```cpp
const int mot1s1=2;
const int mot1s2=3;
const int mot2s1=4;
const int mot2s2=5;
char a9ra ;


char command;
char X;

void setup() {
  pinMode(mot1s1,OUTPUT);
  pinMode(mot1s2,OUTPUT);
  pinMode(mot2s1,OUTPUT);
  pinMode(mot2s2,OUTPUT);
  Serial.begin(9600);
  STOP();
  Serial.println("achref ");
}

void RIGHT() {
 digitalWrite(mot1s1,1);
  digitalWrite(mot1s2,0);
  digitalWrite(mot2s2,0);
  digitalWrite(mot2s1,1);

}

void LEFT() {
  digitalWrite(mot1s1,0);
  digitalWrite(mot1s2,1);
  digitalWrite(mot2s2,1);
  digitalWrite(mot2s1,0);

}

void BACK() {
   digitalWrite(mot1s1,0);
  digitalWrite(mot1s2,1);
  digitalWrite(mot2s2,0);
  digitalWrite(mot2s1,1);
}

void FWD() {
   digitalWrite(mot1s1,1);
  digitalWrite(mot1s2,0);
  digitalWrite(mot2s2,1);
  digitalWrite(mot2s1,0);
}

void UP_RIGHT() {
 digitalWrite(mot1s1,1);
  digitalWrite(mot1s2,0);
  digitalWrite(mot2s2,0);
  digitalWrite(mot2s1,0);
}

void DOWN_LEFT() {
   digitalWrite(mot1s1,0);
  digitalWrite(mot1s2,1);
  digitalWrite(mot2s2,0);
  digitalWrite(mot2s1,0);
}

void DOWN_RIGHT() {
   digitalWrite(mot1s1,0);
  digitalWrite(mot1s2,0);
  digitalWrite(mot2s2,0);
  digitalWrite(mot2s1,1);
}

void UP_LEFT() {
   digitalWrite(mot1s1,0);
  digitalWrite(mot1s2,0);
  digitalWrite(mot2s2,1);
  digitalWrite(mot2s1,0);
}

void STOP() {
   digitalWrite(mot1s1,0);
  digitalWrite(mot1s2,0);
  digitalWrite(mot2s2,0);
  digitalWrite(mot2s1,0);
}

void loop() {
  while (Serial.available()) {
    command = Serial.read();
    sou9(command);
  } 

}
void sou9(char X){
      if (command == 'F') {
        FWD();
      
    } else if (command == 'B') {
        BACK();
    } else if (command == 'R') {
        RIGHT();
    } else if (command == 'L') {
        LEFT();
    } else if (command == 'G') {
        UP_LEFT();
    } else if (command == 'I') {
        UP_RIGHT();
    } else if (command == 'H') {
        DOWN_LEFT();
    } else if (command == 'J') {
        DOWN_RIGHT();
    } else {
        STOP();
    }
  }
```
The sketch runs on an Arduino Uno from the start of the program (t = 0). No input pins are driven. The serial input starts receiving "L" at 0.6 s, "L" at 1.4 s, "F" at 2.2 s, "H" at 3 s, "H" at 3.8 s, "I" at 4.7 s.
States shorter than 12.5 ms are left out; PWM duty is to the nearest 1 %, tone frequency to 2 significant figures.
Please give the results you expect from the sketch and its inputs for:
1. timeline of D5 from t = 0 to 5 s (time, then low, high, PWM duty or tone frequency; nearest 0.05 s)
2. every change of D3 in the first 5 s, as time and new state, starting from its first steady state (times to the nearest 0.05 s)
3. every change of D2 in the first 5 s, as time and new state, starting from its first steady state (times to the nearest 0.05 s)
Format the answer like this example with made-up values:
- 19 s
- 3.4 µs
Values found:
- 0 s low; 0.6 s high; 3 s low
- 0 s low; 0.6 s high; 2.2 s low; 3 s high; 4.7 s low
- 0 s low; 2.2 s high; 3 s low; 4.7 s high
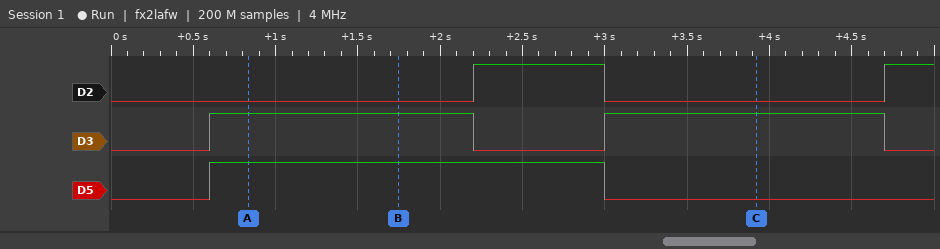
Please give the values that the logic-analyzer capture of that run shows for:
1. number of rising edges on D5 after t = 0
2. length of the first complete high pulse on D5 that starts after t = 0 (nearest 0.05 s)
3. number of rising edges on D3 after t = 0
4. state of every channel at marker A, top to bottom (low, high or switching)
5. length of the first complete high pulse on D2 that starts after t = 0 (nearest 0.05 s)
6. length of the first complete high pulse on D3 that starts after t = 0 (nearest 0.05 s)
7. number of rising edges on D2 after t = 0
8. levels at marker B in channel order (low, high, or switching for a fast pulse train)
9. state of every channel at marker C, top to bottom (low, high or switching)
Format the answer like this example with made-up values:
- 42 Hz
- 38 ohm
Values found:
- 1
- 2.40 s
- 2
- D2 low, D3 high, D5 high
- 0.80 s
- 1.60 s
- 2
- D2 low, D3 high, D5 high
- D2 low, D3 high, D5 low
